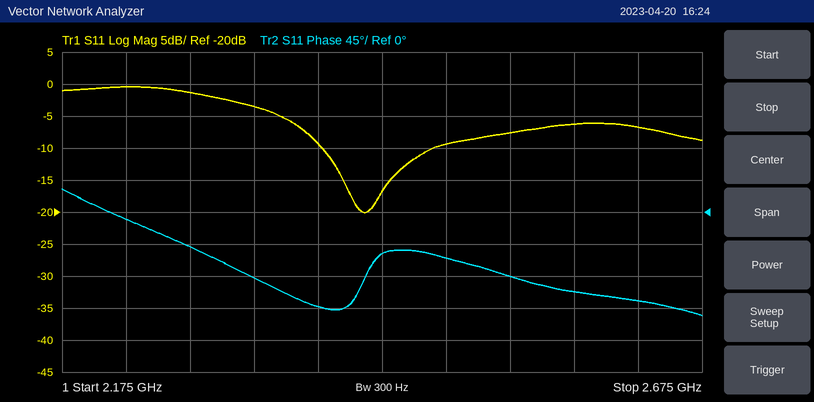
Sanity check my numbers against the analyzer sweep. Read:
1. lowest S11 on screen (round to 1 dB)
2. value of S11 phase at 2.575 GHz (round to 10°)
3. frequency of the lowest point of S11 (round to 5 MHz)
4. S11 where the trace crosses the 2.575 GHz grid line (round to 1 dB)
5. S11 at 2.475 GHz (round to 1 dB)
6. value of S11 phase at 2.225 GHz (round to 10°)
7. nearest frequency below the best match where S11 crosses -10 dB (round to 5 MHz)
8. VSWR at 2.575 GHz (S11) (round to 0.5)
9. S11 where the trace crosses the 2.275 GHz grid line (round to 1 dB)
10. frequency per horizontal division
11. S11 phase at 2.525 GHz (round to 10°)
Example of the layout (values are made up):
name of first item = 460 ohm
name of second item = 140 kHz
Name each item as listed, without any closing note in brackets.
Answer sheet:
lowest S11 on screen = -20 dB
value of S11 phase at 2.575 GHz = -110°
frequency of the lowest point of S11 = 2.410 GHz
S11 where the trace crosses the 2.575 GHz grid line = -6 dB
S11 at 2.475 GHz = -9 dB
value of S11 phase at 2.225 GHz = -10°
nearest frequency below the best match where S11 crosses -10 dB = 2.380 GHz
VSWR at 2.575 GHz (S11) = 3.0
S11 where the trace crosses the 2.275 GHz grid line = -1 dB
frequency per horizontal division = 50 MHz
S11 phase at 2.525 GHz = -90°
